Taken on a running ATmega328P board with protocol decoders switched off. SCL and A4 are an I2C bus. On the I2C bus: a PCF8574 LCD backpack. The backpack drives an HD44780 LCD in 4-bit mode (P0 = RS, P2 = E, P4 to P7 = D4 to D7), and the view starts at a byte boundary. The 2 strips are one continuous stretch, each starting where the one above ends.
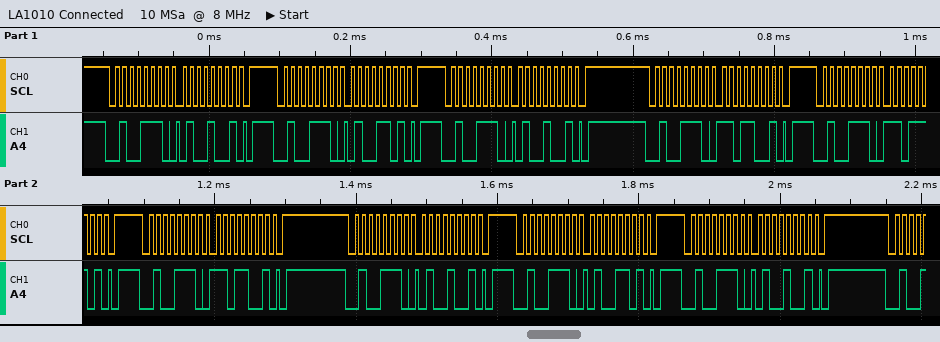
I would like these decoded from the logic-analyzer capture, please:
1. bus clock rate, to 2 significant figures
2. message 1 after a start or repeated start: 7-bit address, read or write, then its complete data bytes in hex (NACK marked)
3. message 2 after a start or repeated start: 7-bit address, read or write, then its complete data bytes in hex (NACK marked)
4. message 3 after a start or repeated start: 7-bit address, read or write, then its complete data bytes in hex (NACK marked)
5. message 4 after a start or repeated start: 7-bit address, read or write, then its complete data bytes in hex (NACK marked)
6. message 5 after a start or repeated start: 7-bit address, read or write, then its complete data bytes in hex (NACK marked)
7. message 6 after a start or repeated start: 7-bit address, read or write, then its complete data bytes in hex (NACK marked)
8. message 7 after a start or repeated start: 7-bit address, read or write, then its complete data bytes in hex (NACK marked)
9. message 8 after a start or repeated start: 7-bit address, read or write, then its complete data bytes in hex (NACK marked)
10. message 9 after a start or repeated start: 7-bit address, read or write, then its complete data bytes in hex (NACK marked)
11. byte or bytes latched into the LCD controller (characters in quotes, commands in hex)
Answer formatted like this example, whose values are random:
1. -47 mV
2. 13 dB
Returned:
1. 100 kHz
2. 0x27 write: 49
3. 0x27 write: 4D
4. 0x27 write: 49
5. 0x27 write: D9
6. 0x27 write: DD
7. 0x27 write: D9
8. 0x27 write: 49
9. 0x27 write: 4D
10. 0x27 write: 49
11. 'M'
